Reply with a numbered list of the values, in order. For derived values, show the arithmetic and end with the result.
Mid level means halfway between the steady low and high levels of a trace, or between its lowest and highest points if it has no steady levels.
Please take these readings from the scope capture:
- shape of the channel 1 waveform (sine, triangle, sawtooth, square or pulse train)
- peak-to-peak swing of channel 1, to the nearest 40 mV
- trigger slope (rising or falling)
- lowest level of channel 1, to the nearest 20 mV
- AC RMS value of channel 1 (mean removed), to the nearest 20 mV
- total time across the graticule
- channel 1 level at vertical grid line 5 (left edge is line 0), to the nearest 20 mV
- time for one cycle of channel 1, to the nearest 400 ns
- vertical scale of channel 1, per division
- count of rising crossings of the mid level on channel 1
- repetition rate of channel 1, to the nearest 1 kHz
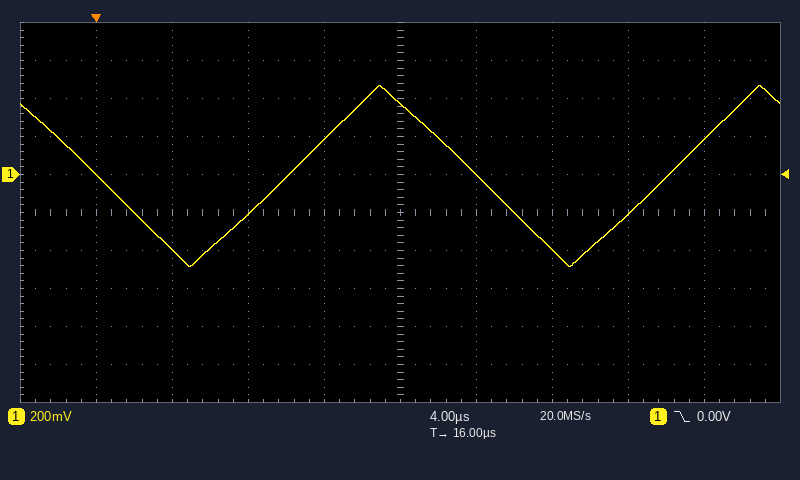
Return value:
1. triangle
2. 960 mV
3. falling
4. -480 mV
5. 960 mV / (2√3) ≈ 277 mV, so 280 mV to the nearest 20 mV
6. 40 µs
7. 380 mV
8. 20.0 µs
9. 200 mV
10. 2
11. 1 / 20.0 µs ≈ 50 kHz
